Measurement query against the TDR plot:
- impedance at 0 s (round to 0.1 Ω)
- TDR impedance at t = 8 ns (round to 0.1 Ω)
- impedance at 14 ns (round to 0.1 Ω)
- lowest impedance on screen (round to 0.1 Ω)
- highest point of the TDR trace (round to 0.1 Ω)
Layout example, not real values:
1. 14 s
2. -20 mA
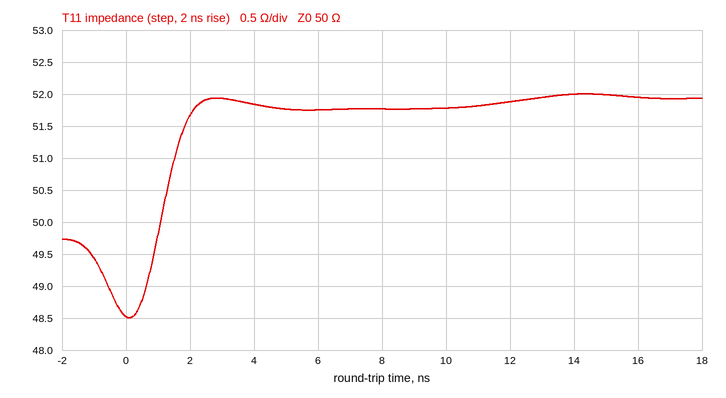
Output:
1. 48.5 Ω
2. 51.8 Ω
3. 52.0 Ω
4. 48.5 Ω
5. 52.0 Ω
